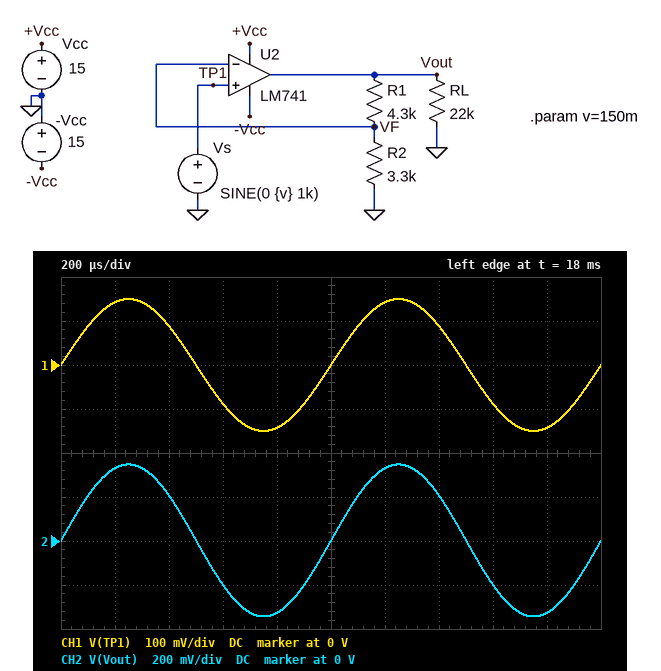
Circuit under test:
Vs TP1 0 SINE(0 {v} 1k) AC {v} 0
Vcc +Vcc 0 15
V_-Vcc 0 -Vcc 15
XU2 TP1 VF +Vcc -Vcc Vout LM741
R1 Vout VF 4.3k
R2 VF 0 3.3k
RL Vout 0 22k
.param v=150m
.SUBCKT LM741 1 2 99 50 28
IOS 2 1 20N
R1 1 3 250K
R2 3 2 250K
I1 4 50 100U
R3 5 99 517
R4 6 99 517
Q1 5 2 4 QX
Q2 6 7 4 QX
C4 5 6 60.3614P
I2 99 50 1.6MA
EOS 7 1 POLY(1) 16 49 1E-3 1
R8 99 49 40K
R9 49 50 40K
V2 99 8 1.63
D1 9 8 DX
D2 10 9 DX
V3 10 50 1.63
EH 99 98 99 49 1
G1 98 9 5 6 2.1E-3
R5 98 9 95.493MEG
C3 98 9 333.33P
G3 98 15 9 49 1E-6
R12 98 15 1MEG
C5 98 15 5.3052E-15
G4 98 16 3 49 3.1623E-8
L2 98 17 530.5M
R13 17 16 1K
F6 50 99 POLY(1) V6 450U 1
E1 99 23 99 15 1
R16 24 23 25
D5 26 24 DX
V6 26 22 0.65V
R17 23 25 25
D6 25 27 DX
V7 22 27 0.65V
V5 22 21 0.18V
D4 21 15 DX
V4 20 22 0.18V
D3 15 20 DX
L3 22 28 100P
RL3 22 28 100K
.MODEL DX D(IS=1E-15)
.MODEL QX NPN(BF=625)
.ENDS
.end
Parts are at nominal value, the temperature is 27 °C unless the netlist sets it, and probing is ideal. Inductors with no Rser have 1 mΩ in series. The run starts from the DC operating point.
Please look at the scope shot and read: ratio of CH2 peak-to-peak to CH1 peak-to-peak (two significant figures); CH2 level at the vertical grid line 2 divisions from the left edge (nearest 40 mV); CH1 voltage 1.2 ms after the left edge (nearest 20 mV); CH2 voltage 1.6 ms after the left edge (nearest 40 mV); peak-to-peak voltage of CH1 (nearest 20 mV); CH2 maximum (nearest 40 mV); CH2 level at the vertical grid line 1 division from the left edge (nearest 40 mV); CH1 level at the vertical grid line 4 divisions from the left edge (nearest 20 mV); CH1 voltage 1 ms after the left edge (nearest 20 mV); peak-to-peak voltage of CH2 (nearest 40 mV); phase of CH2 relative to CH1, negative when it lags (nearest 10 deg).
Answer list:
2.3
200 mV
140 mV
-200 mV
300 mV
360 mV
320 mV
-140 mV
0 V
680 mV
0 deg
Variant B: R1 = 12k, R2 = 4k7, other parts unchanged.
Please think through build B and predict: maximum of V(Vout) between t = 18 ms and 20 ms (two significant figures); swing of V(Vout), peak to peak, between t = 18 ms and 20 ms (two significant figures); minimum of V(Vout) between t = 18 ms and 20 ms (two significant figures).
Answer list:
540 mV
1.1 V
-530 mV
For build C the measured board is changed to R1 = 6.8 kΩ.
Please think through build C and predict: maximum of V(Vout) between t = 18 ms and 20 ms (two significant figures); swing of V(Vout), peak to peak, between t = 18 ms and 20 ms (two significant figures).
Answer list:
460 mV
920 mV
